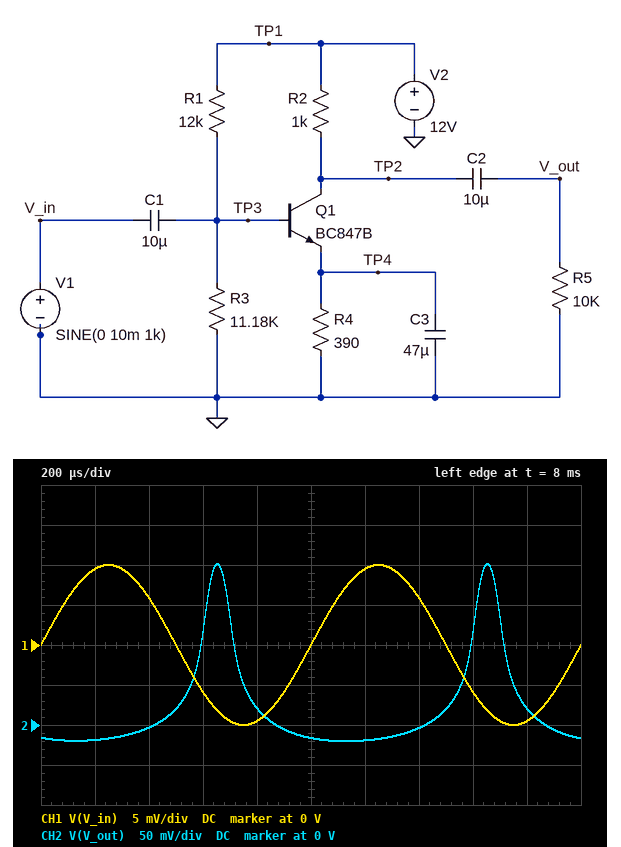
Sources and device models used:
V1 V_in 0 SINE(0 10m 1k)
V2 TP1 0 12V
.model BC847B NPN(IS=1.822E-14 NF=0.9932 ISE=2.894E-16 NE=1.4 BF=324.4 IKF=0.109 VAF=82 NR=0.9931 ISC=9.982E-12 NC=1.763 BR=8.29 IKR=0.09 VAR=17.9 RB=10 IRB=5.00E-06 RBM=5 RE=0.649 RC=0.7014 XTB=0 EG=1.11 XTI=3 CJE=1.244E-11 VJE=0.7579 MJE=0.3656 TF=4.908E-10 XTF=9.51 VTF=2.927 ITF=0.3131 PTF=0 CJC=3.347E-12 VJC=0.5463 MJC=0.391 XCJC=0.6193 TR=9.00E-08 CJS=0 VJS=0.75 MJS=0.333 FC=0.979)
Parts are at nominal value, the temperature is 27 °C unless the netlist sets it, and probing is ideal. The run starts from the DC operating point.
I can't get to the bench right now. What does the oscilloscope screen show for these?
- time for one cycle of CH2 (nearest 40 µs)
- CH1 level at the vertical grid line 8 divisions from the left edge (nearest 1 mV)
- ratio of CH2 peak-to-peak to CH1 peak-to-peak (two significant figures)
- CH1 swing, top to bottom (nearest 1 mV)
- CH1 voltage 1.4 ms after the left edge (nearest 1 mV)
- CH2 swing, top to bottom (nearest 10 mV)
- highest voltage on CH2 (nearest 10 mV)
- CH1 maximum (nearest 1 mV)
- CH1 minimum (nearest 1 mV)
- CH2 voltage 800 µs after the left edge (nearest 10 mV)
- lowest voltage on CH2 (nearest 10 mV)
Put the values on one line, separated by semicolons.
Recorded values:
1.00 ms; -6 mV; 11; 20 mV; 6 mV; 220 mV; 200 mV; 10 mV; -10 mV; 20 mV; -20 mV
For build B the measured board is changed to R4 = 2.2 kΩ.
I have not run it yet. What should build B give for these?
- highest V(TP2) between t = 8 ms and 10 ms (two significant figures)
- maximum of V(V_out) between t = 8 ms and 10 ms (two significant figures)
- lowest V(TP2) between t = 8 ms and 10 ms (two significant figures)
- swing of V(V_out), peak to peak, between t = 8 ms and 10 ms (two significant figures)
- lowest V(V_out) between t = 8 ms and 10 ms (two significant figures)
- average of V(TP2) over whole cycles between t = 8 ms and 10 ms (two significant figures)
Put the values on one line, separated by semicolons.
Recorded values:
10 V; 650 mV; 8.9 V; 1.4 V; -750 mV; 9.7 V
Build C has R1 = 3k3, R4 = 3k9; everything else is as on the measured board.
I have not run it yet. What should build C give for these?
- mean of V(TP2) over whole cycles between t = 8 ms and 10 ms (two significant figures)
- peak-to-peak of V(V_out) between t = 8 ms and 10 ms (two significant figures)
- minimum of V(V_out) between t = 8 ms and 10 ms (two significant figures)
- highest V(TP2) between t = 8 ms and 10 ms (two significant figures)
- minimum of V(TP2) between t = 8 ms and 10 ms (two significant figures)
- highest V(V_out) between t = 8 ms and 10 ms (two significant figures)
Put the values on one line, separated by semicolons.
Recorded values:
9.8 V; 1.3 V; -720 mV; 10 V; 9.1 V; 620 mV
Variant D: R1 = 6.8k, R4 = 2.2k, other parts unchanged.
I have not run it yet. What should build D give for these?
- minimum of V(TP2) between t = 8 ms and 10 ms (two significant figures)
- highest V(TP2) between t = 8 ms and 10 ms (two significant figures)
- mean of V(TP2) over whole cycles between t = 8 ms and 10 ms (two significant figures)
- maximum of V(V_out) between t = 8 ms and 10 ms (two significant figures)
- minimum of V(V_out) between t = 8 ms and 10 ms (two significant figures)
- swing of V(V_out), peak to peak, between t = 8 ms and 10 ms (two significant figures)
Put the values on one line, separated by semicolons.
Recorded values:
8.0 V; 9.8 V; 8.9 V; 820 mV; -940 mV; 1.8 V
